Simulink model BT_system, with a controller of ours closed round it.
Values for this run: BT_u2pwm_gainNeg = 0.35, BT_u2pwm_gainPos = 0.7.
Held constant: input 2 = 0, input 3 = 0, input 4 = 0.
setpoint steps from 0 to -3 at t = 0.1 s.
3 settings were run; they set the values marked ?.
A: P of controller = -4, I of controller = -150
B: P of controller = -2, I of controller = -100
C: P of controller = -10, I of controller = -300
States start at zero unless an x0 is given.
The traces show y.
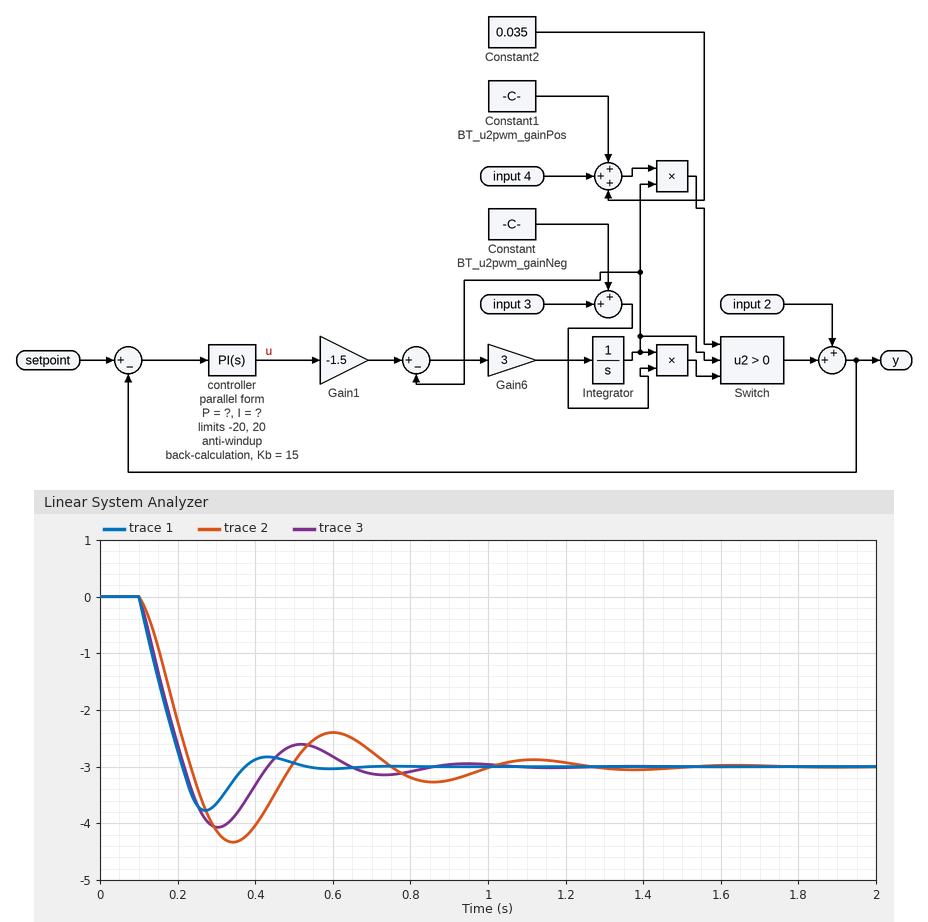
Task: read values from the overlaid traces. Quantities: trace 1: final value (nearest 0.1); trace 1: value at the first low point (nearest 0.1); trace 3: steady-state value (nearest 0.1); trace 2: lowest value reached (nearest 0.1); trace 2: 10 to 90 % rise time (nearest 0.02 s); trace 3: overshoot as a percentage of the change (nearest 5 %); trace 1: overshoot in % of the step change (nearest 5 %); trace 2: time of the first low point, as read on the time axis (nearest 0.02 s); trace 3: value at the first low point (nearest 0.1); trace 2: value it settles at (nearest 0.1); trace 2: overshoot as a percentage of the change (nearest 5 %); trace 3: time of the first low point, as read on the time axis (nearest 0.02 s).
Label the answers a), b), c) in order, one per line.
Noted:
a) -3.0
b) -3.8
c) -3.0
d) -4.3
e) 0.10 s
f) 35 %
g) 25 %
h) 0.34 s
i) -4.1
j) -3.0
k) 45 %
l) 0.30 s
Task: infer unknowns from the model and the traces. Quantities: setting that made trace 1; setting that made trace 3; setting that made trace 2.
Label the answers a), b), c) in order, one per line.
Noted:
a) C
b) A
c) B
